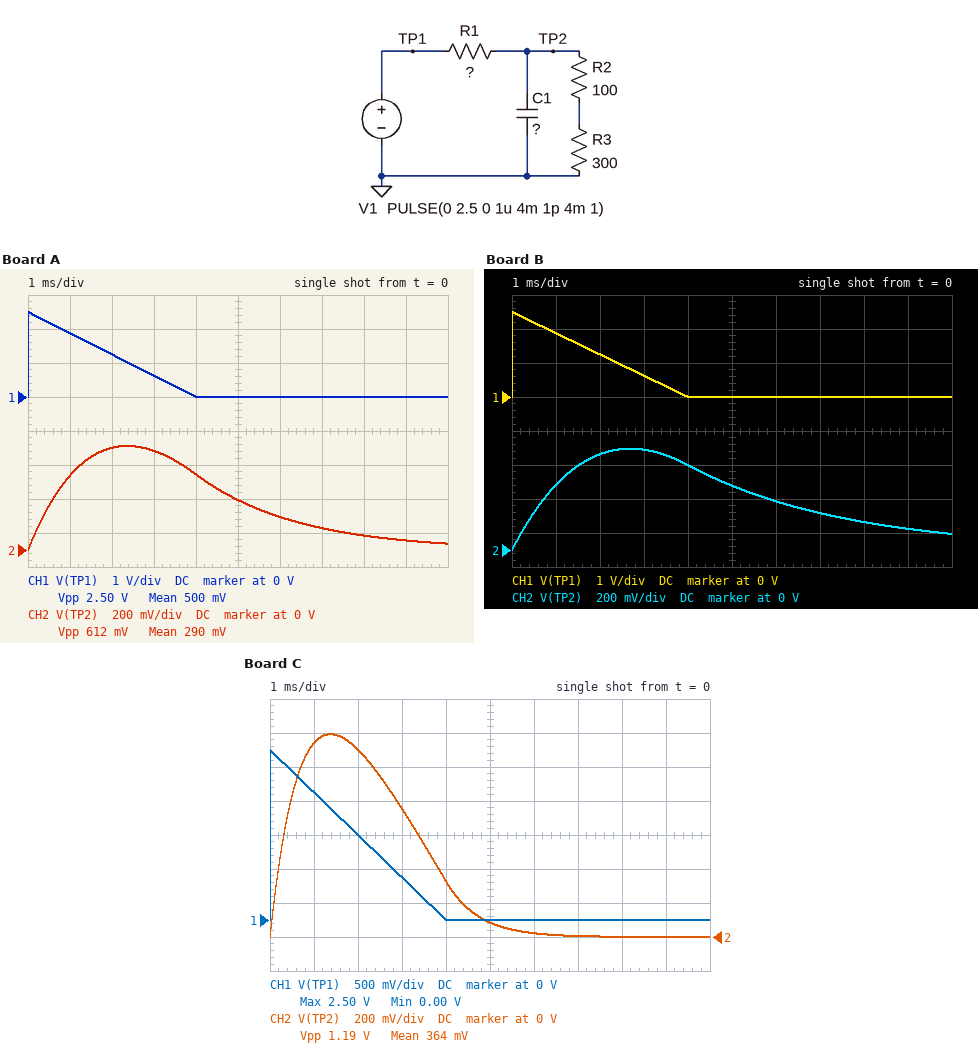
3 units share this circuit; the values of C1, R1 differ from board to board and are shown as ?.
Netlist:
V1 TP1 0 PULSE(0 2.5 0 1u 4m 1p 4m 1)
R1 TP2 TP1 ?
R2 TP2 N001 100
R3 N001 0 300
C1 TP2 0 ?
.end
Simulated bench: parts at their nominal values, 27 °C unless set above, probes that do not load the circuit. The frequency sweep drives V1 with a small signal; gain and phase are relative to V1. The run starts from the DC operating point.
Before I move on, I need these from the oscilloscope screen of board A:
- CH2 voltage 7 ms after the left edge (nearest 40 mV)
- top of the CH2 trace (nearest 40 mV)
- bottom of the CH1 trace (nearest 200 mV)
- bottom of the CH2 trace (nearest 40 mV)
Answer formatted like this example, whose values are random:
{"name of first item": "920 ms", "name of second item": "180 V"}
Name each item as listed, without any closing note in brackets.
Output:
{"CH2 voltage 7 ms after the left edge": "120 mV", "top of the CH2 trace": "600 mV", "bottom of the CH1 trace": "0 V", "bottom of the CH2 trace": "0 V"}
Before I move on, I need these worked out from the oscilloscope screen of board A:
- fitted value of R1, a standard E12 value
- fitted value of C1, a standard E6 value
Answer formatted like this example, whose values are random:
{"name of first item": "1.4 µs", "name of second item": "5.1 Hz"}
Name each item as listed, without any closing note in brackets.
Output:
{"fitted value of R1, a standard E12 value": "270 Ω", "fitted value of C1, a standard E6 value": "15 µF"}
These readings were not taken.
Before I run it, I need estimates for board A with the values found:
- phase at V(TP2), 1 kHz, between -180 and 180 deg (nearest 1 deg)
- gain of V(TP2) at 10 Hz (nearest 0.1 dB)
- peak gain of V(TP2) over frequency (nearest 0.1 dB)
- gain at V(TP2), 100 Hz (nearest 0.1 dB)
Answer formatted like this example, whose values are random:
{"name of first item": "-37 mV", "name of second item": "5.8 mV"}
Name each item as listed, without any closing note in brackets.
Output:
{"phase at V(TP2), 1 kHz, between -180 and 180 deg": "-86 deg", "gain of V(TP2) at 10 Hz": "-4.6 dB", "peak gain of V(TP2) over frequency": "-4.5 dB", "gain at V(TP2), 100 Hz": "-9.7 dB"}
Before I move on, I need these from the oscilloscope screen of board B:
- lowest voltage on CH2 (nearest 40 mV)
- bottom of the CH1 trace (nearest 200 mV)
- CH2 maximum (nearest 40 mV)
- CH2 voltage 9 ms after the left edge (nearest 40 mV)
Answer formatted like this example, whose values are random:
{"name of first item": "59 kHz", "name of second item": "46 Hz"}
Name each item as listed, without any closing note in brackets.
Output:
{"lowest voltage on CH2": "0 V", "bottom of the CH1 trace": "0 V", "CH2 maximum": "600 mV", "CH2 voltage 9 ms after the left edge": "120 mV"}
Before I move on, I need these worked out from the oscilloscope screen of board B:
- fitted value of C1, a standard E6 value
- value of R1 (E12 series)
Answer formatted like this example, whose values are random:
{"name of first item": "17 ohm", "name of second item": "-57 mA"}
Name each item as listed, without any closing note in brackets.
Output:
{"fitted value of C1, a standard E6 value": "33 µF", "value of R1": "150 Ω"}
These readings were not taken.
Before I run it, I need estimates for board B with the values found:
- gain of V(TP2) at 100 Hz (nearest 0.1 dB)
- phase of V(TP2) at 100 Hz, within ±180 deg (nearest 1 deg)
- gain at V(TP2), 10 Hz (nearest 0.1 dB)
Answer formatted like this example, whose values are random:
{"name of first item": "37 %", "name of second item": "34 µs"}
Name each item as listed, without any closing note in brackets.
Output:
{"gain of V(TP2) at 100 Hz": "-10.6 dB", "phase of V(TP2) at 100 Hz, within ±180 deg": "-66 deg", "gain at V(TP2), 10 Hz": "-3.0 dB"}
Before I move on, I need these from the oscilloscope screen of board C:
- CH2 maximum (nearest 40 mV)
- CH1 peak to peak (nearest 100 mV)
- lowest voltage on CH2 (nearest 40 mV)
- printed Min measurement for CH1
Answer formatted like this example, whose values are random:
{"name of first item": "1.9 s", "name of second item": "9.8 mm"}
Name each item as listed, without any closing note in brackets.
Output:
{"CH2 maximum": "1.20 V", "CH1 peak to peak": "2.5 V", "lowest voltage on CH2": "0 V", "printed Min measurement for CH1": "0.00 V"}
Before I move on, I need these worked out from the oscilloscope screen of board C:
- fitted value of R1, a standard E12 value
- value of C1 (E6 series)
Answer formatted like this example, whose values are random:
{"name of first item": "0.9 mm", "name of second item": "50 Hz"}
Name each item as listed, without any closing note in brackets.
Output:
{"fitted value of R1, a standard E12 value": "150 Ω", "value of C1": "6.8 µF"}
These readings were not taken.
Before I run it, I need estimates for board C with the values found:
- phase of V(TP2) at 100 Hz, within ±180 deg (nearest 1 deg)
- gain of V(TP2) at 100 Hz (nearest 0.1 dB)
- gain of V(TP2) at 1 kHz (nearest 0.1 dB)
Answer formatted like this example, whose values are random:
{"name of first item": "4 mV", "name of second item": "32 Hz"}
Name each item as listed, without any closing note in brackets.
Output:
{"phase of V(TP2) at 100 Hz, within ±180 deg": "-25 deg", "gain of V(TP2) at 100 Hz": "-3.6 dB", "gain of V(TP2) at 1 kHz": "-16.3 dB"}
